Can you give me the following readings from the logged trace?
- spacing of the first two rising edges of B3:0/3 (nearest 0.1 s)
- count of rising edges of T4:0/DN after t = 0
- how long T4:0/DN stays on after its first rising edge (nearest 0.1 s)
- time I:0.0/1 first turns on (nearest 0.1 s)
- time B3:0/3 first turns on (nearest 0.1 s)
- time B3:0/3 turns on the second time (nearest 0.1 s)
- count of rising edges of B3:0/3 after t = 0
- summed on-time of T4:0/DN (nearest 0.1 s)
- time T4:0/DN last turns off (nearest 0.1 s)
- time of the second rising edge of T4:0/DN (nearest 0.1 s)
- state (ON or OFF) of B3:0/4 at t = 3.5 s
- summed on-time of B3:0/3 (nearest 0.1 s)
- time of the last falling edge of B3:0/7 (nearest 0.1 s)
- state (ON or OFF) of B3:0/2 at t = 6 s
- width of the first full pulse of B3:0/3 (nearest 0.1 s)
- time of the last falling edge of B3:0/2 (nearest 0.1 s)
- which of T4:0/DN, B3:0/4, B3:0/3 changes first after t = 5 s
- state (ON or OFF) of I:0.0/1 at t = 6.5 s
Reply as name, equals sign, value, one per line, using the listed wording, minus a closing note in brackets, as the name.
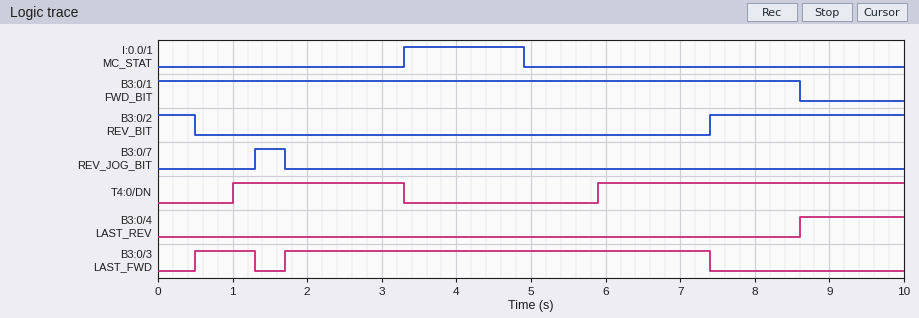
spacing of the first two rising edges of B3:0/3 = 1.2 s
count of rising edges of T4:0/DN after t = 0 = 2
how long T4:0/DN stays on after its first rising edge = 2.3 s
time I:0.0/1 first turns on = 3.3 s
time B3:0/3 first turns on = 0.5 s
time B3:0/3 turns on the second time = 1.7 s
count of rising edges of B3:0/3 after t = 0 = 2
summed on-time of T4:0/DN = 6.4 s
time T4:0/DN last turns off = 3.3 s
time of the second rising edge of T4:0/DN = 5.9 s
state (ON or OFF) of B3:0/4 at t = 3.5 s = OFF
summed on-time of B3:0/3 = 6.5 s
time of the last falling edge of B3:0/7 = 1.7 s
state (ON or OFF) of B3:0/2 at t = 6 s = OFF
width of the first full pulse of B3:0/3 = 0.8 s
time of the last falling edge of B3:0/2 = 0.5 s
which of T4:0/DN, B3:0/4, B3:0/3 changes first after t = 5 s = T4:0/DN
state (ON or OFF) of I:0.0/1 at t = 6.5 s = OFF
